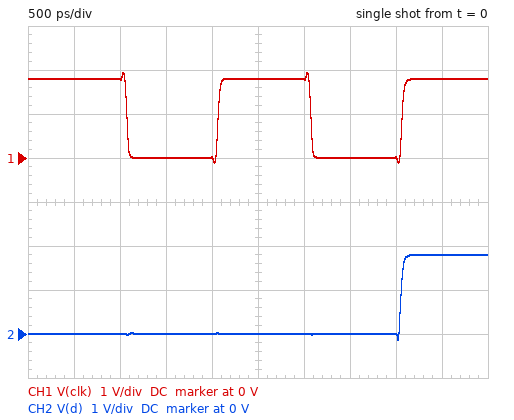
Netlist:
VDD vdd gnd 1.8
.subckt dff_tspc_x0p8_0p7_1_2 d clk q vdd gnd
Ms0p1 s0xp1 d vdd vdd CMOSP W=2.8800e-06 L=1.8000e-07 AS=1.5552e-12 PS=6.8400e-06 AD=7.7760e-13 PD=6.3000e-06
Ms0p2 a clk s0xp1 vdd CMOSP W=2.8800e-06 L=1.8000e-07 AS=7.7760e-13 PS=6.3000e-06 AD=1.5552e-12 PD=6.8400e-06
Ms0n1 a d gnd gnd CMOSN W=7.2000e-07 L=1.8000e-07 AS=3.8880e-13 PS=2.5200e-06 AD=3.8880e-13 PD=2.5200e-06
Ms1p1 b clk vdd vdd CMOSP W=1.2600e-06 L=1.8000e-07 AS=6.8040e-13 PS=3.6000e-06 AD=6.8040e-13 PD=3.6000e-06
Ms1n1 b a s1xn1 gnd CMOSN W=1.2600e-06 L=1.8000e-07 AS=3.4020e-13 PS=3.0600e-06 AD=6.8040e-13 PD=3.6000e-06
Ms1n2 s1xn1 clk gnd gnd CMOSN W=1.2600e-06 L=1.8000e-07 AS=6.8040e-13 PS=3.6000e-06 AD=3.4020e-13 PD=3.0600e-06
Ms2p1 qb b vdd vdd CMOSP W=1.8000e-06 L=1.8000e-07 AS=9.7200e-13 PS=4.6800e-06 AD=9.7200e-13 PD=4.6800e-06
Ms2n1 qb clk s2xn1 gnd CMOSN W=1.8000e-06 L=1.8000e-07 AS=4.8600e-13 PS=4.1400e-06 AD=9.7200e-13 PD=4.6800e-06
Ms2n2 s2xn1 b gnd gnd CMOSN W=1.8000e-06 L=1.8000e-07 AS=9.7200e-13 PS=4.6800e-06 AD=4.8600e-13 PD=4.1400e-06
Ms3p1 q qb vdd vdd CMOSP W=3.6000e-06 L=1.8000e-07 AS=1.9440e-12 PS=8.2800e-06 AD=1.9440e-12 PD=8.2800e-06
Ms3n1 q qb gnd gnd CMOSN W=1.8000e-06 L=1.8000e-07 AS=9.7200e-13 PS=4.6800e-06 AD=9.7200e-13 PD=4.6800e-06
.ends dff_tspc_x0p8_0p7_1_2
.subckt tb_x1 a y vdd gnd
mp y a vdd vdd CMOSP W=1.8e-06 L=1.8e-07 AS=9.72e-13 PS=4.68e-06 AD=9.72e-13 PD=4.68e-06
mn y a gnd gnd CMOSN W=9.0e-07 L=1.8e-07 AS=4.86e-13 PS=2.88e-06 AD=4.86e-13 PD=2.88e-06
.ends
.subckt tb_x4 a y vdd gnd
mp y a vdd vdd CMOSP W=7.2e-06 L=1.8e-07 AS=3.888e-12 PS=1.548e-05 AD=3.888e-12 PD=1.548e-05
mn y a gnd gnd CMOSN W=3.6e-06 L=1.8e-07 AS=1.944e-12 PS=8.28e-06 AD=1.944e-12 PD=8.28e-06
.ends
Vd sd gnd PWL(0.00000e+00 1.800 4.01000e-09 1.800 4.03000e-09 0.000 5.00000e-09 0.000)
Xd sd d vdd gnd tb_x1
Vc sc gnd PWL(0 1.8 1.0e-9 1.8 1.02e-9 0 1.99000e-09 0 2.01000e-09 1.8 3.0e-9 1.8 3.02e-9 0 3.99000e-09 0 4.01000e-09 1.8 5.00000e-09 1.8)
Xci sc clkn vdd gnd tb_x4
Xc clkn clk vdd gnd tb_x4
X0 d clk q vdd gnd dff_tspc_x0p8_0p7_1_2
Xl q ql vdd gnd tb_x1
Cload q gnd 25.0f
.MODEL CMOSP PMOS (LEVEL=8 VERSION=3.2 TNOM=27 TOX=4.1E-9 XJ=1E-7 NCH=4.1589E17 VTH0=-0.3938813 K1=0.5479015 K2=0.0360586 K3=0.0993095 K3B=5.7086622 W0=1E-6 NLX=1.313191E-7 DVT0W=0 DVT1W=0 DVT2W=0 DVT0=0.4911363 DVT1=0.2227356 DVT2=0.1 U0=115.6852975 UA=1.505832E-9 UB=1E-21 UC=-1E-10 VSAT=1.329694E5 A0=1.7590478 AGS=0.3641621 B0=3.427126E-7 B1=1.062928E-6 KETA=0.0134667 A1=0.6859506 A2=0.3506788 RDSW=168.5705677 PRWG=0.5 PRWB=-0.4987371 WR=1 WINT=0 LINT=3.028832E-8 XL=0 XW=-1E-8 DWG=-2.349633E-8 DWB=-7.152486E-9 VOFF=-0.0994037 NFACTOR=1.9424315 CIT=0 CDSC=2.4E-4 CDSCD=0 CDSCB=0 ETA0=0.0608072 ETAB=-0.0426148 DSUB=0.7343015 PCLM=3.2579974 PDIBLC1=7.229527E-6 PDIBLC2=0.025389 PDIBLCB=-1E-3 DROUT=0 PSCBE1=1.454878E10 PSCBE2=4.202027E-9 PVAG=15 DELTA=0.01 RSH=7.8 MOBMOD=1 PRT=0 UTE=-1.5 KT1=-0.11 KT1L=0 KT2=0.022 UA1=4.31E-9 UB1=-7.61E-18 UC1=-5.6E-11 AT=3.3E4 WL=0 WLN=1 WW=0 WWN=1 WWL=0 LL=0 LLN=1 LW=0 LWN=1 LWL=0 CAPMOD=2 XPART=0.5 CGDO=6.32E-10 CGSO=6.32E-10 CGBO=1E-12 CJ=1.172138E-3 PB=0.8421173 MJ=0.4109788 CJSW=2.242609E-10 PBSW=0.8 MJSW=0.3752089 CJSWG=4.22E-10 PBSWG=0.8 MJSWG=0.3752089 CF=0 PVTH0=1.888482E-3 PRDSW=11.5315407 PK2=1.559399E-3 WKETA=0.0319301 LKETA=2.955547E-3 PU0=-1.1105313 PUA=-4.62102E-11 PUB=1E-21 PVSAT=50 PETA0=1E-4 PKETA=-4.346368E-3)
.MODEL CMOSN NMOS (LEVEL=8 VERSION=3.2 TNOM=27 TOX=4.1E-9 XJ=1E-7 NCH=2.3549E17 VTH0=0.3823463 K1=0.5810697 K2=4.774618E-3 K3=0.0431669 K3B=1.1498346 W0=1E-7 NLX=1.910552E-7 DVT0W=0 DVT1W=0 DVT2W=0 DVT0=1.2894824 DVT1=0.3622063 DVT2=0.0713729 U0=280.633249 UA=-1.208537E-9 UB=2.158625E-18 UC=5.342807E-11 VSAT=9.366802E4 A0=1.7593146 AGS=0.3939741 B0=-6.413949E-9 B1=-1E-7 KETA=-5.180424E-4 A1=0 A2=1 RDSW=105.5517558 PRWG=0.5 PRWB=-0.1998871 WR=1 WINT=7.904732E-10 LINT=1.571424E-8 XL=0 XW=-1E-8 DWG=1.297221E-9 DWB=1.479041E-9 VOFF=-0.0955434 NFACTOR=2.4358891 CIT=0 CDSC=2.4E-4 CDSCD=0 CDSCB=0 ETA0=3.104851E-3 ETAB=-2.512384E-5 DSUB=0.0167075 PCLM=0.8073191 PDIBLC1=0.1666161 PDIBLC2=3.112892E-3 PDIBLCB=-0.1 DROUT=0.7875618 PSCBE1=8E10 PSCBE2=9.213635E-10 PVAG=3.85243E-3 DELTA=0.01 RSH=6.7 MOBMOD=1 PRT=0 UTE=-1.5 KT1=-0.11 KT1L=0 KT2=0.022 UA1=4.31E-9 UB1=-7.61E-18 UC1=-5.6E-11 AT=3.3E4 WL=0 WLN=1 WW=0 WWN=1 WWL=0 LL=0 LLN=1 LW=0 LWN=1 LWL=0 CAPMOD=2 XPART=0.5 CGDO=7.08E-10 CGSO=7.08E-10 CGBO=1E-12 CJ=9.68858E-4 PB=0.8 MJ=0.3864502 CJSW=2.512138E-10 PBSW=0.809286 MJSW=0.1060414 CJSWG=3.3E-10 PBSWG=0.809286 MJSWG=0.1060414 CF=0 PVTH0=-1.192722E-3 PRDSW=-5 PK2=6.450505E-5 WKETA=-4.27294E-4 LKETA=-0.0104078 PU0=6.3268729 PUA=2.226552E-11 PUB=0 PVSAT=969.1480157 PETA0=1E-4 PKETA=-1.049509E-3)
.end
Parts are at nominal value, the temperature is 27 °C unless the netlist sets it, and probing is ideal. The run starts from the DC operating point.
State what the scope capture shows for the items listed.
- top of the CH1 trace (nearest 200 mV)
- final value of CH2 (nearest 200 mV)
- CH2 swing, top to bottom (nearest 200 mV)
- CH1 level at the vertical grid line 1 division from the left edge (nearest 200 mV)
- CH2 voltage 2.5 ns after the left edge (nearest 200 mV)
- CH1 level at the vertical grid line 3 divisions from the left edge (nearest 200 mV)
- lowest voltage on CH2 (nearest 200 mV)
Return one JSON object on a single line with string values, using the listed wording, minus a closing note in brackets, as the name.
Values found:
{"top of the CH1 trace": "2.0 V", "final value of CH2": "1.8 V", "CH2 swing, top to bottom": "2.0 V", "CH1 level at the vertical grid line 1 division from the left edge": "1.8 V", "CH2 voltage 2.5 ns after the left edge": "0 V", "CH1 level at the vertical grid line 3 divisions from the left edge": "0 V", "lowest voltage on CH2": "-200 mV"}
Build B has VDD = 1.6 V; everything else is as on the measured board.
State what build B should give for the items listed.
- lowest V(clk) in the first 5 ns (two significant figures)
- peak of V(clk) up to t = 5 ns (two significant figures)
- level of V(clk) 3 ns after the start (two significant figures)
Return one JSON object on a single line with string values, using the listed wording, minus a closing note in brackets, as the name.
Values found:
{"lowest V(clk) in the first 5 ns": "-130 mV", "peak of V(clk) up to t = 5 ns": "1.7 V", "level of V(clk) 3 ns after the start": "1.6 V"}
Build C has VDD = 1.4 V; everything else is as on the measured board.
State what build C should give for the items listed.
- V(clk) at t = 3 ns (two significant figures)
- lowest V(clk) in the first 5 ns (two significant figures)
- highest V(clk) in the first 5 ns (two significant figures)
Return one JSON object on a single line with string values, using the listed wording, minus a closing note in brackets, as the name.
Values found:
{"V(clk) at t = 3 ns": "1.4 V", "lowest V(clk) in the first 5 ns": "-150 mV", "highest V(clk) in the first 5 ns": "1.5 V"}
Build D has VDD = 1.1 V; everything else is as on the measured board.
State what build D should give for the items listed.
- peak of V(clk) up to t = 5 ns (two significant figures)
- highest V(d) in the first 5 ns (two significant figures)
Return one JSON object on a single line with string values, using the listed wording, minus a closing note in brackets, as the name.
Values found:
{"peak of V(clk) up to t = 5 ns": "1.2 V", "highest V(d) in the first 5 ns": "1.1 V"}
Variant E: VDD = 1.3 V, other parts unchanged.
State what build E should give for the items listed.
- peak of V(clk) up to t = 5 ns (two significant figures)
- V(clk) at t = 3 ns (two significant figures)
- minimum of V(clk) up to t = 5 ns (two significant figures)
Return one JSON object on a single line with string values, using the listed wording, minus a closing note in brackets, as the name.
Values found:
{"peak of V(clk) up to t = 5 ns": "1.4 V", "V(clk) at t = 3 ns": "1.3 V", "minimum of V(clk) up to t = 5 ns": "-170 mV"}
